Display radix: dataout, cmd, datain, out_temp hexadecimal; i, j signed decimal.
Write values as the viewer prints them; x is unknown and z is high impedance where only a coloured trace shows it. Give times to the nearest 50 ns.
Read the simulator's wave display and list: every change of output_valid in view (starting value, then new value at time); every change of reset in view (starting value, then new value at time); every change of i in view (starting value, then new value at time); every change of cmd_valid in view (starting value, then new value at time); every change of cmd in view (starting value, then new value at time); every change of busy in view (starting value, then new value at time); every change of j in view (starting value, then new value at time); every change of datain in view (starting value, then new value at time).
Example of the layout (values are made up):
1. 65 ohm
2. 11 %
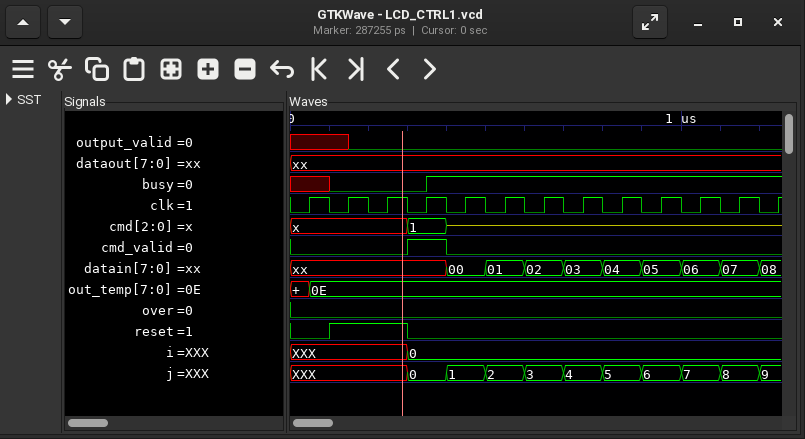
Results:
1. x, 0 at 150 ns
2. 0, 1 at 100 ns, 0 at 300 ns
3. XXX, 0 at 300 ns
4. 0, 1 at 300 ns, 0 at 400 ns
5. x, 1 at 300 ns, z at 400 ns
6. x, 0 at 100 ns, 1 at 350 ns
7. XXX, 0 at 300 ns, 1 at 400 ns, 2 at 500 ns, 3 at 600 ns, 4 at 700 ns, 5 at 800 ns, 6 at 900 ns, 7 at 1000 ns, 8 at 1100 ns, 9 at 1200 ns
8. xx, 00 at 400 ns, 01 at 500 ns, 02 at 600 ns, 03 at 700 ns, 04 at 800 ns, 05 at 900 ns, 06 at 1000 ns, 07 at 1100 ns, 08 at 1200 ns
